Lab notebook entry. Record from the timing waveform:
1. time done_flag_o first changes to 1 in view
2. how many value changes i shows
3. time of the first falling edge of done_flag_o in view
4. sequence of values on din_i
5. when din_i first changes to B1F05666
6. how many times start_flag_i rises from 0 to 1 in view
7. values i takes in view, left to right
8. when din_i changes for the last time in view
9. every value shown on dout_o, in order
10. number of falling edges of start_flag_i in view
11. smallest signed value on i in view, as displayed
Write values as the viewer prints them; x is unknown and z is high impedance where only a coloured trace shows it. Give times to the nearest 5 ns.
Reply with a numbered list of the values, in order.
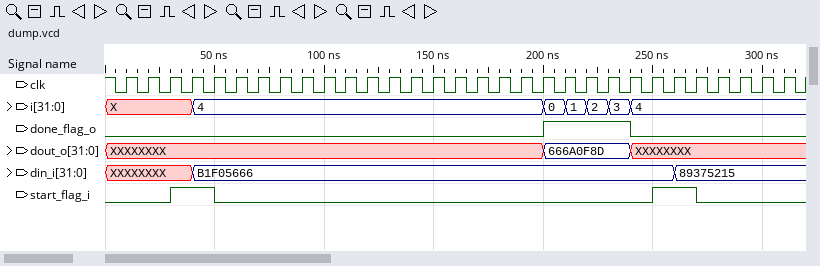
1. 200 ns
2. 6
3. 240 ns
4. XXXXXXXX, B1F05666, 89375215
5. 40 ns
6. 2
7. X, 4, 0, 1, 2, 3, 4
8. 260 ns
9. XXXXXXXX, 666A0F8D, XXXXXXXX
10. 2
11. 0
